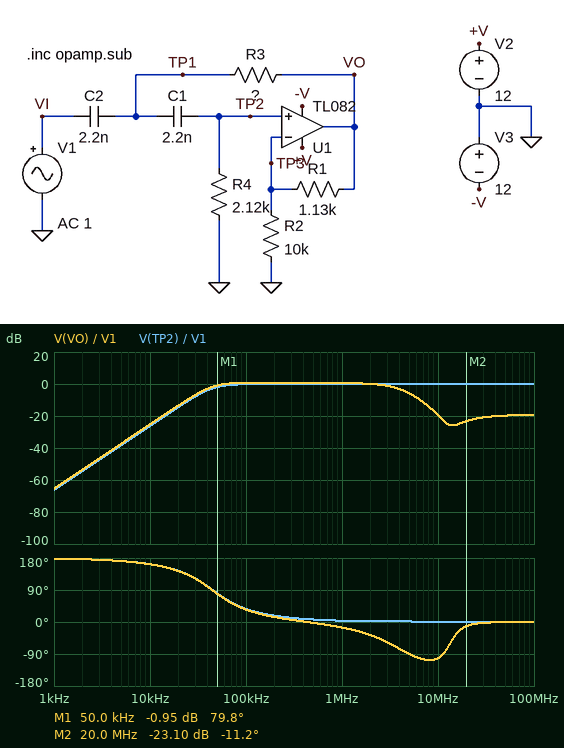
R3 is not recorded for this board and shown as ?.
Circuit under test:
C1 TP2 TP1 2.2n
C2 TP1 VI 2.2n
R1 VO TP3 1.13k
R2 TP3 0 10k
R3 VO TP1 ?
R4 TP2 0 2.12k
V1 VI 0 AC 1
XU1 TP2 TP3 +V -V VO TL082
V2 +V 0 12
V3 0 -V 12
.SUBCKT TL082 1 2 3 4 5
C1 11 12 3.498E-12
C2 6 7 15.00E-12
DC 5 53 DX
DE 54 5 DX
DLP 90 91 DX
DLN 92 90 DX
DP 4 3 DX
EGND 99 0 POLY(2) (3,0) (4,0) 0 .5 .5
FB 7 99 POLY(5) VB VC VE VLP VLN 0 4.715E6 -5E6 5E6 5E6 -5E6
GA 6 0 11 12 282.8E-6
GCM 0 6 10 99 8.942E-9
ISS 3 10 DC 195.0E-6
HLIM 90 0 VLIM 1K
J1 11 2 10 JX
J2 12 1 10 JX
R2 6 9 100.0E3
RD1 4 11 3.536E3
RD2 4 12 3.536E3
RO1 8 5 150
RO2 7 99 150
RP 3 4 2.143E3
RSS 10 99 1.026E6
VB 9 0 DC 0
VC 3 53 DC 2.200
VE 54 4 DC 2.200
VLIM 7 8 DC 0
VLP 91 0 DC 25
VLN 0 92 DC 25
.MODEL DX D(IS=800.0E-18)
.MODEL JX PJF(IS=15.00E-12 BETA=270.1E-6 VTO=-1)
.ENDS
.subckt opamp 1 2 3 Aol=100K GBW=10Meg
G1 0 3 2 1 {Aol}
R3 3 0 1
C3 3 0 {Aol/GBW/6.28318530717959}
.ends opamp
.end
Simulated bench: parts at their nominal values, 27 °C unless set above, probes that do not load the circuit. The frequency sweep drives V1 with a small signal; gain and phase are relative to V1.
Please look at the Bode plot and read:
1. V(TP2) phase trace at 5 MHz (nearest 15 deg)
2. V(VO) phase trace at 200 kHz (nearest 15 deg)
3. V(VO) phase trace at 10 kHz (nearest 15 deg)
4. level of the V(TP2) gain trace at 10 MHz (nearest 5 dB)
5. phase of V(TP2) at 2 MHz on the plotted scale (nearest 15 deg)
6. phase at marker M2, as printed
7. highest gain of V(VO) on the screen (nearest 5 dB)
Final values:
0 deg
15 deg
165 deg
0 dB
0 deg
-11.2 deg
0 dB
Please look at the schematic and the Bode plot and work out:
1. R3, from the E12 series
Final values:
1.2 kΩ
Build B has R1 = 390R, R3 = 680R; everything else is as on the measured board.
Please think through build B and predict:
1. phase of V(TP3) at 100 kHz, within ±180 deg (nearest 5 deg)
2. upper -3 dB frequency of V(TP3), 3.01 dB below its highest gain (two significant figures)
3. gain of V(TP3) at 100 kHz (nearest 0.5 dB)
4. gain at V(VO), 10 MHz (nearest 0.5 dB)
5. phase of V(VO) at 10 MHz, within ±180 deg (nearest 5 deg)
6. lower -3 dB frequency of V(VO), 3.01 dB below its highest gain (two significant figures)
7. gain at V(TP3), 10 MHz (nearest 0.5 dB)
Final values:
40 deg
2.9 MHz
0.5 dB
-19.0 dB
-50 deg
51 kHz
-19.5 dB
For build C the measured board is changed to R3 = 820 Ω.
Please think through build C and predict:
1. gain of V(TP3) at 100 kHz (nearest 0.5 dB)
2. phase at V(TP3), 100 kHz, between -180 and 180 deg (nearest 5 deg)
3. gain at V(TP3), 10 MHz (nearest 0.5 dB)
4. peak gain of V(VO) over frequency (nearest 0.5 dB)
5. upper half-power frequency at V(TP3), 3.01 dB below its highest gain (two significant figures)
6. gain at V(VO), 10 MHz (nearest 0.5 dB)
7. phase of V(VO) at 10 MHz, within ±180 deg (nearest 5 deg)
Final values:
0.5 dB
35 deg
-21.0 dB
1.5 dB
2.8 MHz
-20.0 dB
-70 deg
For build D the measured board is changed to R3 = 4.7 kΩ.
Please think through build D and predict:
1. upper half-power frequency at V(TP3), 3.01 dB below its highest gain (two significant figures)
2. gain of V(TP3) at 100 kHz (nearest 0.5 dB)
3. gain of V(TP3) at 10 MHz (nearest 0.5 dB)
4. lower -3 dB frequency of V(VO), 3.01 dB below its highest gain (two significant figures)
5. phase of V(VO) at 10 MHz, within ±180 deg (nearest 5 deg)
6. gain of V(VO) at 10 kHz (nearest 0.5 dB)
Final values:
4.1 MHz
-1.5 dB
-16.0 dB
58 kHz
-135 deg
-17.0 dB
